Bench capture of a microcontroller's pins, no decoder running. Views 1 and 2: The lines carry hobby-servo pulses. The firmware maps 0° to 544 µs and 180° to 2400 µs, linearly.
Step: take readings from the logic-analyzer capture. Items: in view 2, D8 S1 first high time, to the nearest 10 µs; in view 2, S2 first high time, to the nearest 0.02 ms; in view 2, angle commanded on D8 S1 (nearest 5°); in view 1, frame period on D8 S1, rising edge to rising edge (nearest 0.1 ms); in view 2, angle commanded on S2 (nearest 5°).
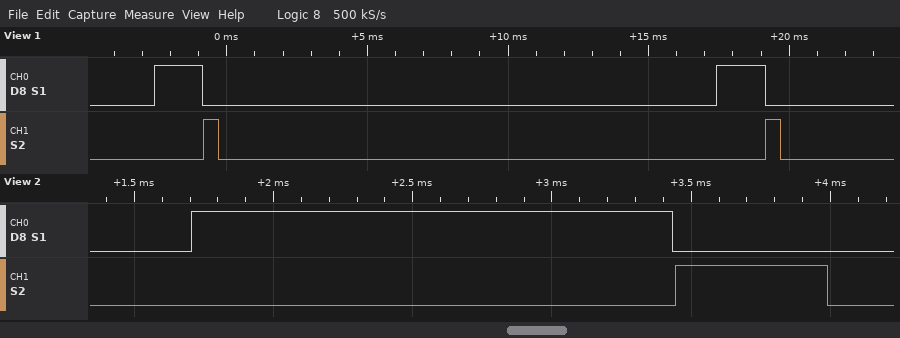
1730 µs
0.54 ms
115°
20.0 ms
0°
